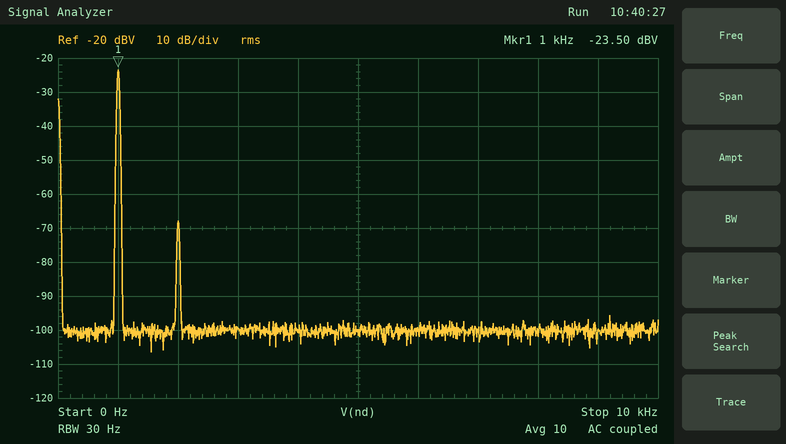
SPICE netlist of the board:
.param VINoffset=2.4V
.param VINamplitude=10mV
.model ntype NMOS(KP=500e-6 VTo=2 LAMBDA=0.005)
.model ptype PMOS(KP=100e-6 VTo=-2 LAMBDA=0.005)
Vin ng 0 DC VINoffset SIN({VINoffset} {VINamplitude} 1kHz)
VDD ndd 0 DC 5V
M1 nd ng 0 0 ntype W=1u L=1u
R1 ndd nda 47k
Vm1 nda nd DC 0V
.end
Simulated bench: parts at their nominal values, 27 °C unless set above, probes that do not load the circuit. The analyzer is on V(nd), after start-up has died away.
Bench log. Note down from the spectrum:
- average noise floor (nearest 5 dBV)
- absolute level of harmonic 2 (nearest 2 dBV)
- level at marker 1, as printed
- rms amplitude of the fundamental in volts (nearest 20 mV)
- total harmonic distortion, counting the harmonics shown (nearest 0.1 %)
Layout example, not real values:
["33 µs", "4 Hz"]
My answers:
["-100 dBV", "-68 dBV", "-23.50 dBV", "60 mV", "0.6 %"]
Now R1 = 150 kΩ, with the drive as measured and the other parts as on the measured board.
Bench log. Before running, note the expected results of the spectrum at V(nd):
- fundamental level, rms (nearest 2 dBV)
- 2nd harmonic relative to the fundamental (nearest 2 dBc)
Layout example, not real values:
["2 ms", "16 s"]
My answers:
["-42 dBV", "-28 dBc"]
